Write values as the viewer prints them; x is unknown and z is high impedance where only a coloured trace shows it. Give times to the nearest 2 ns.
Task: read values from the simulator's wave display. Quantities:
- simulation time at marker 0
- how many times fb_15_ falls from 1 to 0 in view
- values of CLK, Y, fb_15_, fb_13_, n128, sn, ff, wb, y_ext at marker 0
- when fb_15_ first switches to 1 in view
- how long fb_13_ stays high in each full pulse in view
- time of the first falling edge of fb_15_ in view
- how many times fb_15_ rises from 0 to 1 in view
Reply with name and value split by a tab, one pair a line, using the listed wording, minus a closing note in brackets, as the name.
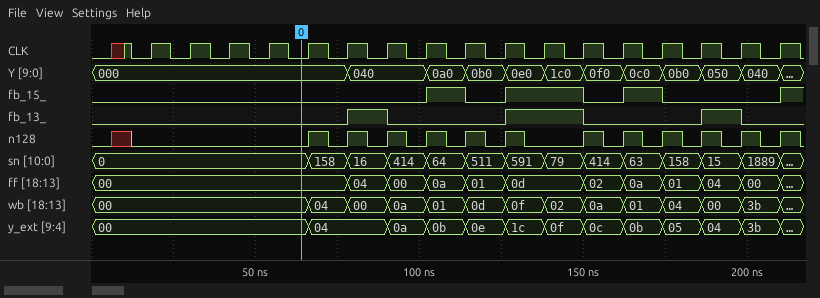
simulation time at marker 0	64 ns
how many times fb_15_ falls from 1 to 0 in view	3
values of CLK, Y, fb_15_, fb_13_, n128, sn, ff, wb, y_ext at marker 0	CLK=0, Y=000, fb_15_=0, fb_13_=0, n128=0, sn=0, ff=00, wb=00, y_ext=00
when fb_15_ first switches to 1 in view	102 ns
how long fb_13_ stays high in each full pulse in view	12 ns, 24 ns, 12 ns
time of the first falling edge of fb_15_ in view	114 ns
how many times fb_15_ rises from 0 to 1 in view	4
